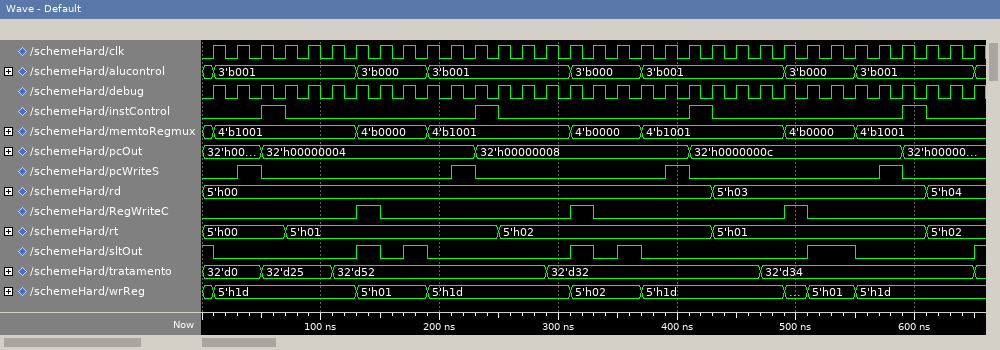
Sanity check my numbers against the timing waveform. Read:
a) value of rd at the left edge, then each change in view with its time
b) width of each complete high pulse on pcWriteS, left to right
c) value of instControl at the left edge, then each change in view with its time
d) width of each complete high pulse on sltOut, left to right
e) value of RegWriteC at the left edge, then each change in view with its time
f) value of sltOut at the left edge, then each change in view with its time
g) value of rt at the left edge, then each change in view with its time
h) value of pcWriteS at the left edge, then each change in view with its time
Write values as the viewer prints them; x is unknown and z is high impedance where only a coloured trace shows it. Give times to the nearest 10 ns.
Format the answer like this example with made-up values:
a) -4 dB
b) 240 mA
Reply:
a) 5'h00, 5'h03 at 430 ns, 5'h04 at 610 ns
b) 20 ns, 20 ns, 20 ns, 20 ns
c) 0, 1 at 50 ns, 0 at 70 ns, 1 at 230 ns, 0 at 250 ns, 1 at 410 ns, 0 at 430 ns, 1 at 590 ns, 0 at 610 ns
d) 20 ns, 20 ns, 20 ns, 20 ns, 40 ns
e) 0, 1 at 130 ns, 0 at 150 ns, 1 at 310 ns, 0 at 330 ns, 1 at 490 ns, 0 at 510 ns
f) 1, 0 at 10 ns, 1 at 130 ns, 0 at 150 ns, 1 at 170 ns, 0 at 190 ns, 1 at 310 ns, 0 at 330 ns, 1 at 350 ns, 0 at 370 ns, 1 at 510 ns, 0 at 550 ns, 1 at 650 ns
g) 5'h00, 5'h01 at 70 ns, 5'h02 at 250 ns, 5'h01 at 430 ns, 5'h02 at 610 ns
h) 0, 1 at 30 ns, 0 at 50 ns, 1 at 210 ns, 0 at 230 ns, 1 at 390 ns, 0 at 410 ns, 1 at 570 ns, 0 at 590 ns
